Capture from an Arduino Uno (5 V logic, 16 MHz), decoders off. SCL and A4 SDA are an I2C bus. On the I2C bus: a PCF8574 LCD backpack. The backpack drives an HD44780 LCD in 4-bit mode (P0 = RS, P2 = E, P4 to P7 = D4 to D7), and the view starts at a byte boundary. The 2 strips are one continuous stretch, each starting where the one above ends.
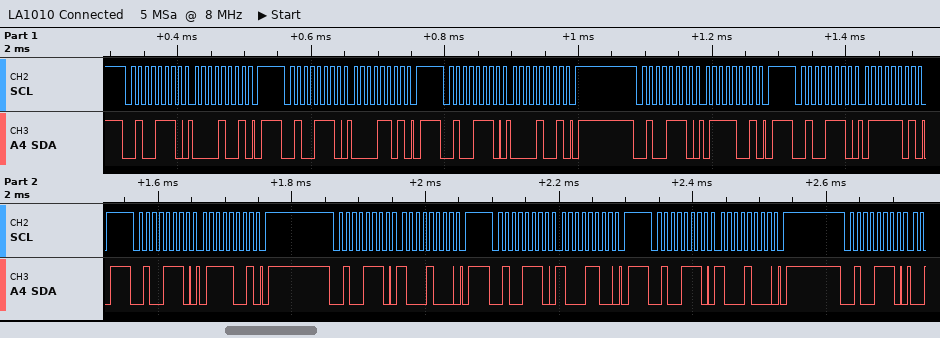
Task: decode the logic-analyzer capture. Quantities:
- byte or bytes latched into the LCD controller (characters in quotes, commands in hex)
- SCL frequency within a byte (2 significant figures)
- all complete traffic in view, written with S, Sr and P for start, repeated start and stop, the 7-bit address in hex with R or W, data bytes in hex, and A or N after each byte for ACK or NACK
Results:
data 0x07
100 kHz
S 27W A 09 A P S 27W A 0D A P S 27W A 09 A P S 27W A 79 A P S 27W A 7D A P S 27W A 79 A P S 27W A 88 A P S 27W A 8C A P S 27W A 88 A P S 27W A
